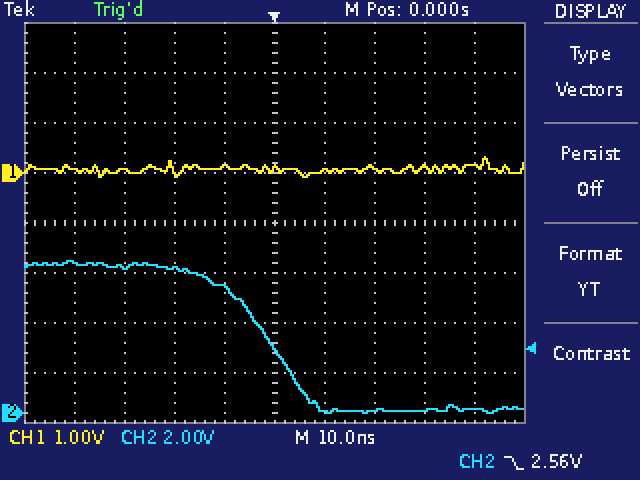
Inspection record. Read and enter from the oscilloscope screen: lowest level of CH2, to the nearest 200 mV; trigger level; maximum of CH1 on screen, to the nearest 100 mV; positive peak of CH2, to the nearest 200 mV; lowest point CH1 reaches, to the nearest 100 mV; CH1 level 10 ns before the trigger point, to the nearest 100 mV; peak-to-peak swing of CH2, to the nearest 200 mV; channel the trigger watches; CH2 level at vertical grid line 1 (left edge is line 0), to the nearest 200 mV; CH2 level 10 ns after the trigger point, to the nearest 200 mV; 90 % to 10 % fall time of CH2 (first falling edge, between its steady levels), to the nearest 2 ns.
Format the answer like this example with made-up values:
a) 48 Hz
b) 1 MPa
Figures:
a) 0.0 V
b) 2.56 V
c) 300 mV
d) 6.0 V
e) -100 mV
f) 100 mV
g) 6.0 V
h) CH2
i) 6.0 V
j) 0.0 V
k) 20 ns
